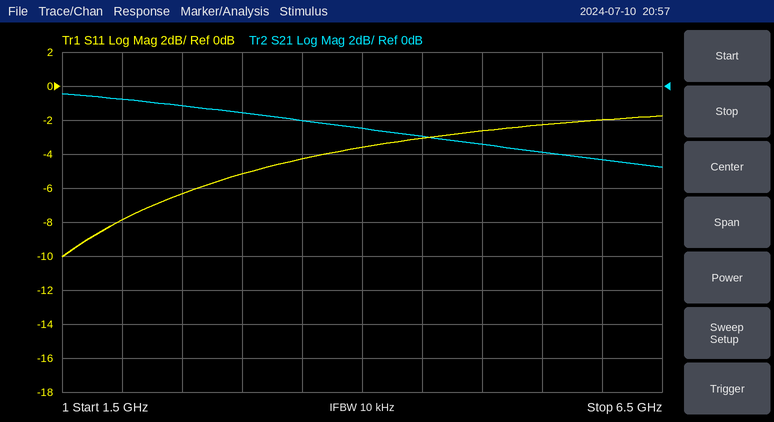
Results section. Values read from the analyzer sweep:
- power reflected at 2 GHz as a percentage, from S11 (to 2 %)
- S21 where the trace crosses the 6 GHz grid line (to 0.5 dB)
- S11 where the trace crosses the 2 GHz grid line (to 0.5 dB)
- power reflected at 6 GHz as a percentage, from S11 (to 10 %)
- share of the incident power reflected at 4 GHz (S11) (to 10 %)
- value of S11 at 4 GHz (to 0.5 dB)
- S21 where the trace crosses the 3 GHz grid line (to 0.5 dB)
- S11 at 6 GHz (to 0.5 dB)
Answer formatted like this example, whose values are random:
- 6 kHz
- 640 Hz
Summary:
- 16 %
- -4.5 dB
- -8.0 dB
- 60 %
- 40 %
- -3.5 dB
- -1.5 dB
- -2.0 dB
